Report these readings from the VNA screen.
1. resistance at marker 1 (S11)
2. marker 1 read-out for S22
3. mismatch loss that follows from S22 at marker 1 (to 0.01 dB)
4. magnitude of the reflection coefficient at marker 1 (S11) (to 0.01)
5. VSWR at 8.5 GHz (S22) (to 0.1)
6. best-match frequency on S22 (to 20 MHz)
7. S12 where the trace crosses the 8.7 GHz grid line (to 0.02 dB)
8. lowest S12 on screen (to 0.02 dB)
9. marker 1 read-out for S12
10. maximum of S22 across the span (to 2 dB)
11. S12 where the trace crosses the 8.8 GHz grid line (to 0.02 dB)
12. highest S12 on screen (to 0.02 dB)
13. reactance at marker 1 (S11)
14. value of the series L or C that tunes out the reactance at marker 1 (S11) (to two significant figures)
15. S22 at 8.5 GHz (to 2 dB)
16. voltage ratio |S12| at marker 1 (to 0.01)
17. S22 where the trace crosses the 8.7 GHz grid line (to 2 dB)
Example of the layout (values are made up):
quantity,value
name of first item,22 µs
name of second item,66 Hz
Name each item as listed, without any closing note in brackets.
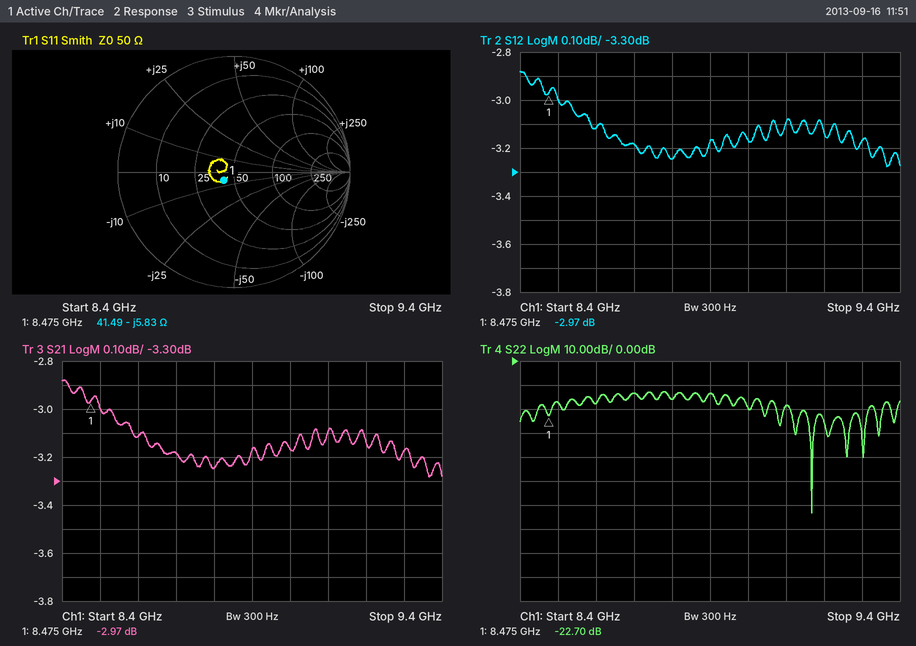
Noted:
quantity,value
resistance at marker 1,41.49 Ω
marker 1 read-out for S22,-22.70 dB
mismatch loss that follows from S22 at marker 1,0.02 dB
magnitude of the reflection coefficient at marker 1 (S11),0.11
VSWR at 8.5 GHz (S22),1.3
best-match frequency on S22,9.16 GHz
S12 where the trace crosses the 8.7 GHz grid line,-3.18 dB
lowest S12 on screen,-3.28 dB
marker 1 read-out for S12,-2.97 dB
maximum of S22 across the span,-12 dB
S12 where the trace crosses the 8.8 GHz grid line,-3.24 dB
highest S12 on screen,-2.88 dB
reactance at marker 1,-5.83 Ω
value of the series L or C that tunes out the reactance at marker 1 (S11),110 pH
S22 at 8.5 GHz,-18 dB
voltage ratio |S12| at marker 1,0.71
S22 where the trace crosses the 8.7 GHz grid line,-14 dB
